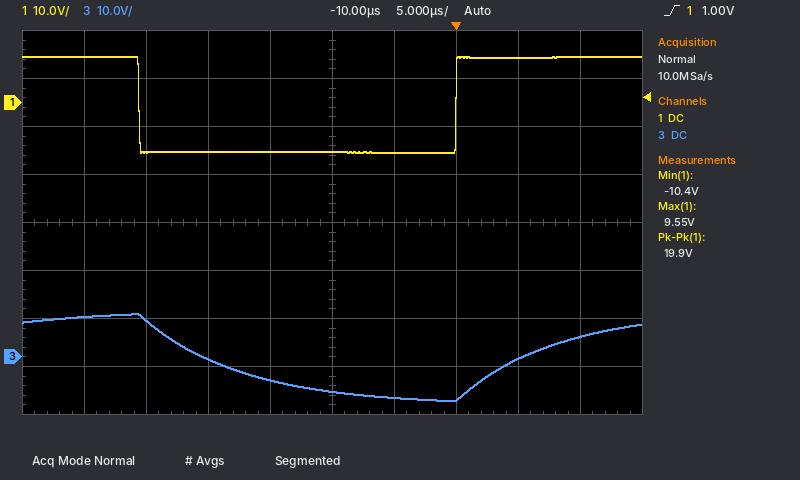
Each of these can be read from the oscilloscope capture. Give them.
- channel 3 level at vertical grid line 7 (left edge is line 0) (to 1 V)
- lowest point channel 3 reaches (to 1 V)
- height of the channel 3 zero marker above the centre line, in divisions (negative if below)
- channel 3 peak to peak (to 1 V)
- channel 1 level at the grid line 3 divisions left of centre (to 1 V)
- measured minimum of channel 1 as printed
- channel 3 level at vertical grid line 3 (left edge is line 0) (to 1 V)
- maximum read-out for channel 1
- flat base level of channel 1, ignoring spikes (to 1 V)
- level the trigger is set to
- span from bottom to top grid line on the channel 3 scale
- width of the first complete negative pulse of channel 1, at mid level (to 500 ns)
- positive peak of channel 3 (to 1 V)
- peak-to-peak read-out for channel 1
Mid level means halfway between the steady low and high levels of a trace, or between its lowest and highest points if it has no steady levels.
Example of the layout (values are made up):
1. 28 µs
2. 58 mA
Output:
1. -9 V
2. -9 V
3. -2.8 div
4. 18 V
5. -10 V
6. -10.4 V
7. 0 V
8. 9.55 V
9. -10 V
10. 1.00 V
11. 80 V
12. 25.5 µs
13. 9 V
14. 19.9 V
